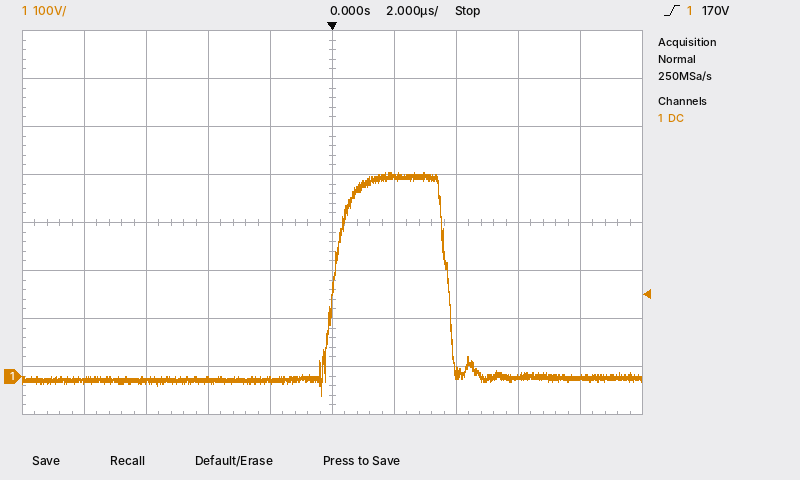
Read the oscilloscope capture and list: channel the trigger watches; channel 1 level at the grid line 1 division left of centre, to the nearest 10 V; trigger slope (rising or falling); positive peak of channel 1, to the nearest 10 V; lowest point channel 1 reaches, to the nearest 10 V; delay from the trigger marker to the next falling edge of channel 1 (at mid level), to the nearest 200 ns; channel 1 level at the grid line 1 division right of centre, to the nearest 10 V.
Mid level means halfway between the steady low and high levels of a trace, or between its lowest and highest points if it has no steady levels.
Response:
channel 1
-10 V
rising
420 V
-40 V
3.8 µs
420 V
